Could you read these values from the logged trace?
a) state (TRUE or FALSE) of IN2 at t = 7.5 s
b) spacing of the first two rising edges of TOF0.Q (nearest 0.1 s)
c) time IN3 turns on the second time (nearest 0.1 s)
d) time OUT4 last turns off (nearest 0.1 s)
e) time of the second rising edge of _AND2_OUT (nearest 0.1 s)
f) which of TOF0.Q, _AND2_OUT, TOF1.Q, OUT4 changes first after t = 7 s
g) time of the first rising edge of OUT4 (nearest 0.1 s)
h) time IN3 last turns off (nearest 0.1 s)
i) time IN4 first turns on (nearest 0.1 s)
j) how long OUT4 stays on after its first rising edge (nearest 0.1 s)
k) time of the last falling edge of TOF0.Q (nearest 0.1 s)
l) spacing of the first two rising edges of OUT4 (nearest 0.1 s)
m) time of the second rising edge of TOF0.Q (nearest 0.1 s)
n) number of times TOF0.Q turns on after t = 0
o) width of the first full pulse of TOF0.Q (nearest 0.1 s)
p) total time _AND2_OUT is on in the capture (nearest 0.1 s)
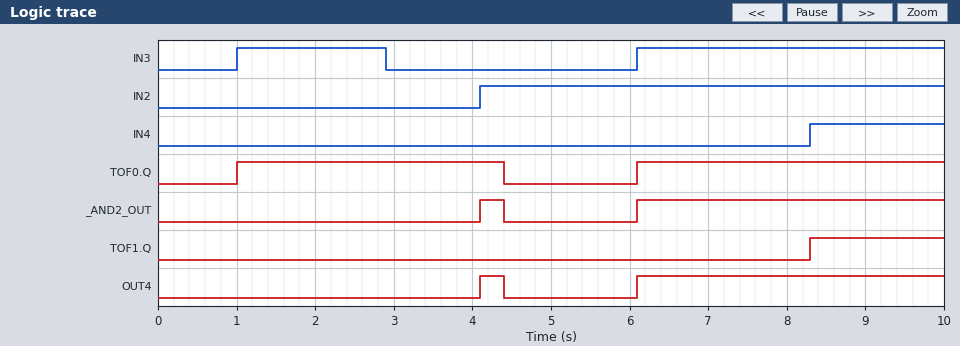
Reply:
TRUE
5.1 s
6.1 s
4.4 s
6.1 s
TOF1.Q
4.1 s
2.9 s
8.3 s
0.3 s
4.4 s
2.0 s
6.1 s
2
3.4 s
4.2 s
